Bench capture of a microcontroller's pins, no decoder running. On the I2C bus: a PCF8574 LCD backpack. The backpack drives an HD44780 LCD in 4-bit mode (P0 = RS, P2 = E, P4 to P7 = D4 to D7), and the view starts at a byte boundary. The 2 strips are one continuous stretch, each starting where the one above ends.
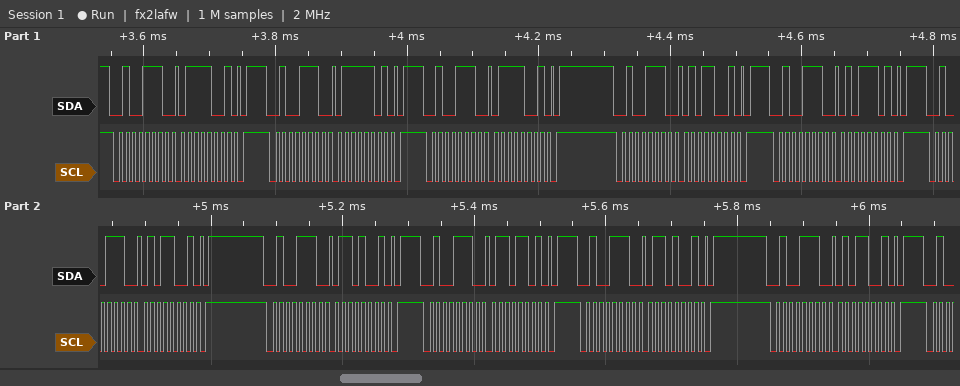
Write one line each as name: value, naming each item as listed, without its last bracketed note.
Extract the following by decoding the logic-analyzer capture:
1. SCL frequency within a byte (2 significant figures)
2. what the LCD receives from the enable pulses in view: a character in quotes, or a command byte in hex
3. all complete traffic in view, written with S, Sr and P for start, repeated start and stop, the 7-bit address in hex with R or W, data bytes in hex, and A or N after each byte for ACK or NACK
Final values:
SCL frequency within a byte: 100 kHz
what the LCD receives from the enable pulses in view: a character in quotes, or a command byte in hex: 'u'
all complete traffic in view, written with S, Sr and P for start, repeated start and stop, the 7-bit address in hex with R or W, data bytes in hex, and A or N after each byte for ACK or NACK: S 27W A 79 A P S 27W A 7D A P S 27W A 79 A P S 27W A 59 A P S 27W A 5D A P S 27W A 59 A P S 27W A 69 A P S 27W A 6D A P S 27W A 69 A P S 27W A 59 A P
